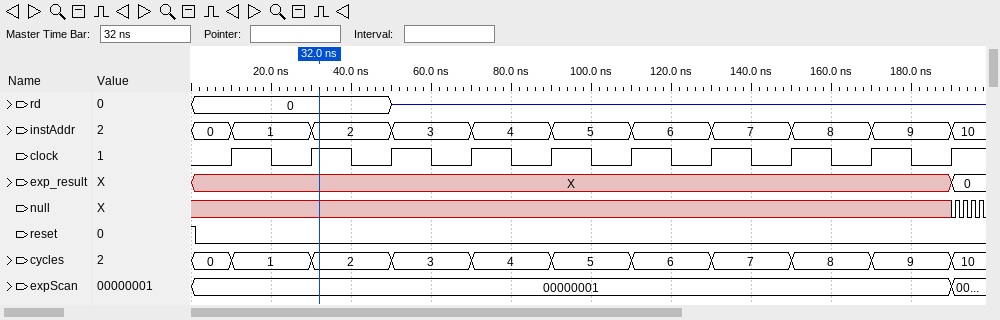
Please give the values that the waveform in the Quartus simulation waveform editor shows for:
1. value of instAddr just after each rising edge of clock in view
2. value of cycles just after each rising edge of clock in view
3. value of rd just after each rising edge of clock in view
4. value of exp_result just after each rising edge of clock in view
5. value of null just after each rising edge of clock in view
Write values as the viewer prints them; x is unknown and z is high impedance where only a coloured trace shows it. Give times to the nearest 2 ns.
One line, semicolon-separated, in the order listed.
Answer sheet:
1, 2, 3, 4, 5, 6, 7, 8, 9, 10; 1, 2, 3, 4, 5, 6, 7, 8, 9, 10; 0, 0, z, z, z, z, z, z, z, z; X, X, X, X, X, X, X, X, X, 0; x x x x x x x x x 0
